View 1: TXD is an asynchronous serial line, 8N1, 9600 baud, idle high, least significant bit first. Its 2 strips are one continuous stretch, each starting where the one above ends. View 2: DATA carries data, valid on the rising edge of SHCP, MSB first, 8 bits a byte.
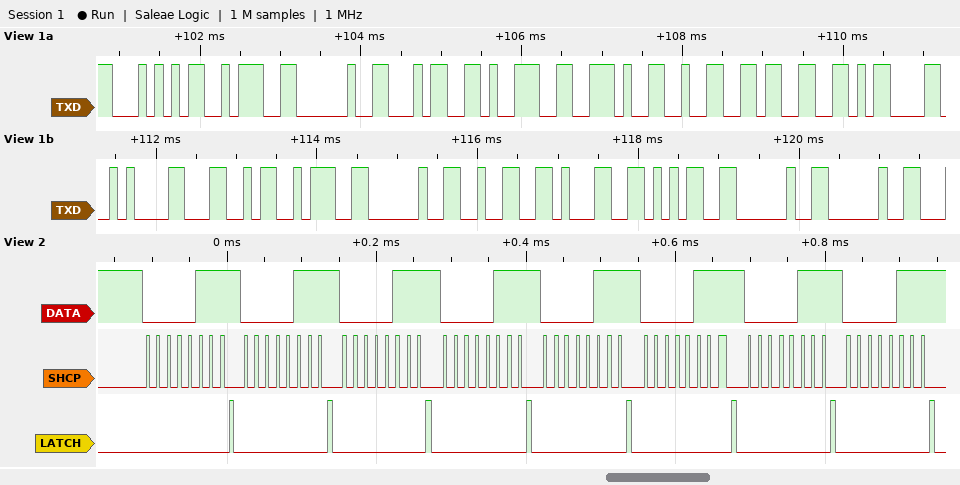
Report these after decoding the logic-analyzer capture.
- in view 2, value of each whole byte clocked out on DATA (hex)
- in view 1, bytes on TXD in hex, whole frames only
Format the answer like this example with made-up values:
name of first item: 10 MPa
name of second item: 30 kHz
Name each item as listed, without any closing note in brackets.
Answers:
in view 2, value of each whole byte clocked out on DATA: 07 07 07 07 07 07 07 07
in view 1, bytes on TXD in hex, whole frames only: 54 3A 20 34 39 2E 32 33 0D 0A 4C 3A 20 32 31 35 20 20
